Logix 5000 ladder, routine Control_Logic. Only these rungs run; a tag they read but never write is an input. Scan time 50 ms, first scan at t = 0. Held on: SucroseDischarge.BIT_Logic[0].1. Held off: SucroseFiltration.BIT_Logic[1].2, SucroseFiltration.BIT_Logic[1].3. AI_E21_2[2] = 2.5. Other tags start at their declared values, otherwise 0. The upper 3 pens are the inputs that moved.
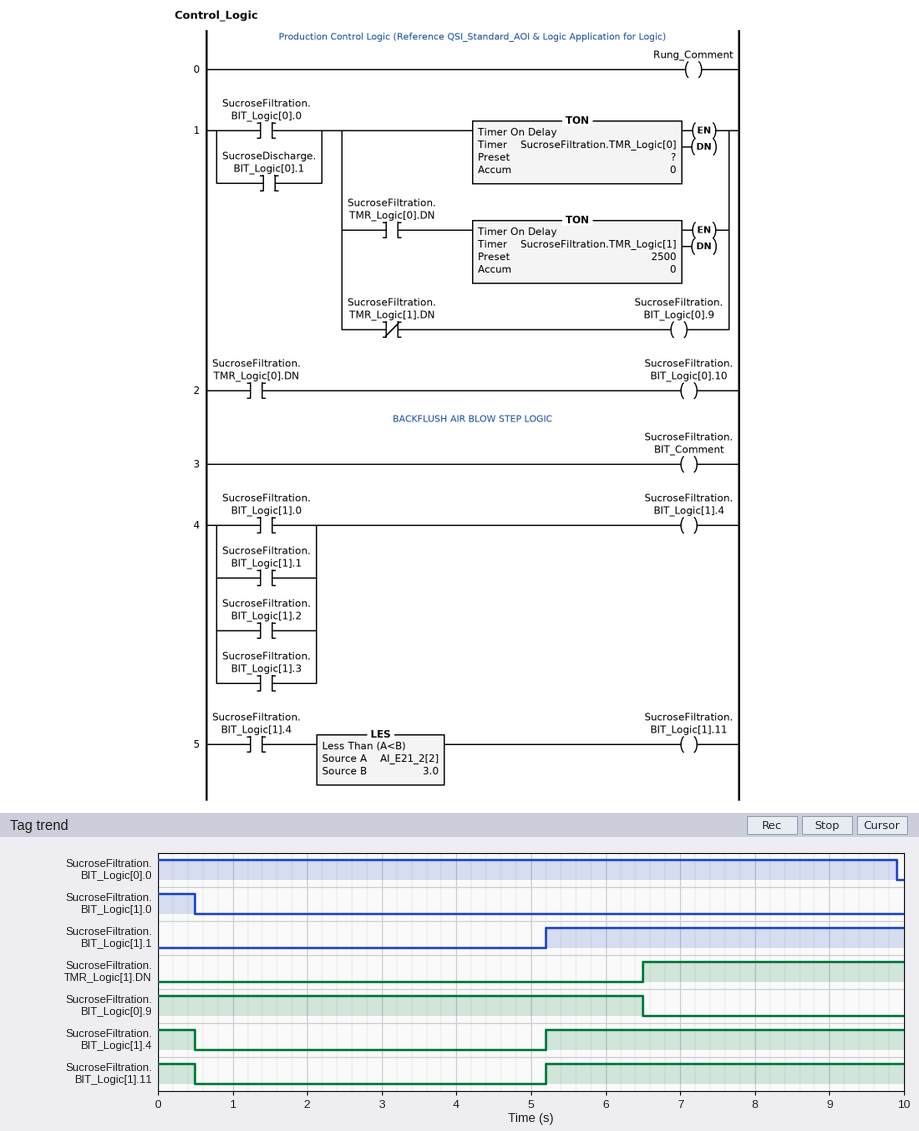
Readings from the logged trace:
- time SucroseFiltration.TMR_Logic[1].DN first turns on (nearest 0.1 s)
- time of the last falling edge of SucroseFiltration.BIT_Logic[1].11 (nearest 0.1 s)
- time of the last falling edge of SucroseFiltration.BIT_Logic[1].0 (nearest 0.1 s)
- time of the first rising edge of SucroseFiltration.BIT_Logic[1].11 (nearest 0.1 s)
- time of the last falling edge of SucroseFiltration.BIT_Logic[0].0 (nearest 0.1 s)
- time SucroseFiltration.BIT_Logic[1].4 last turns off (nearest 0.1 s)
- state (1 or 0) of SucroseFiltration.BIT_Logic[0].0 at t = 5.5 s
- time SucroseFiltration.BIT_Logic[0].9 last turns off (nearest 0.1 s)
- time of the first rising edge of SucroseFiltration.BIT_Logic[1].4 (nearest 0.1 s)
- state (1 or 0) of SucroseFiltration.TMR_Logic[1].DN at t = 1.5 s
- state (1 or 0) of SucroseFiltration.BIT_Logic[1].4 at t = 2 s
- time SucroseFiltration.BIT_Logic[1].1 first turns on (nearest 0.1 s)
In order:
6.5 s
0.5 s
0.5 s
5.2 s
9.9 s
0.5 s
1
6.5 s
5.2 s
0
0
5.2 s
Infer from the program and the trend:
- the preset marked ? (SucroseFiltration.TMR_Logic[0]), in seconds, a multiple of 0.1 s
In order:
4.0 s
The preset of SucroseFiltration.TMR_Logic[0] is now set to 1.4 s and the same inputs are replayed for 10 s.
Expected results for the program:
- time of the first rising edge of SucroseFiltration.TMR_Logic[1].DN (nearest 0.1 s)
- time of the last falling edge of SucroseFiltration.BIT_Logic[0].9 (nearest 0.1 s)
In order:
3.9 s
3.9 s
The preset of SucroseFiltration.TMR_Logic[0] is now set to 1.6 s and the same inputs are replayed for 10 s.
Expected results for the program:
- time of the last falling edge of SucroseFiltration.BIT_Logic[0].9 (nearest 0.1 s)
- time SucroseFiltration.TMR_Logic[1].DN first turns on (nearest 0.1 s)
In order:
4.1 s
4.1 s
